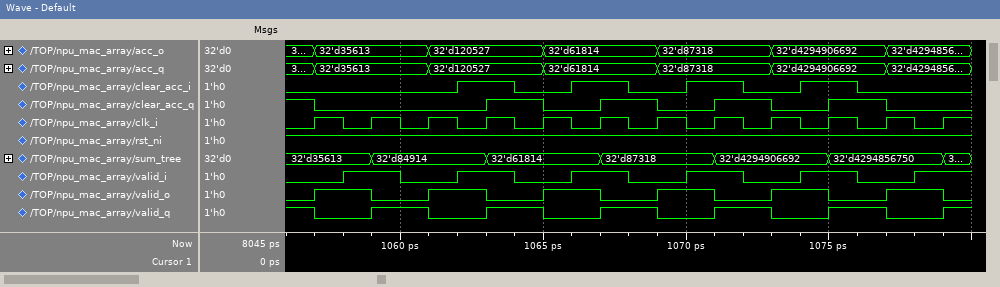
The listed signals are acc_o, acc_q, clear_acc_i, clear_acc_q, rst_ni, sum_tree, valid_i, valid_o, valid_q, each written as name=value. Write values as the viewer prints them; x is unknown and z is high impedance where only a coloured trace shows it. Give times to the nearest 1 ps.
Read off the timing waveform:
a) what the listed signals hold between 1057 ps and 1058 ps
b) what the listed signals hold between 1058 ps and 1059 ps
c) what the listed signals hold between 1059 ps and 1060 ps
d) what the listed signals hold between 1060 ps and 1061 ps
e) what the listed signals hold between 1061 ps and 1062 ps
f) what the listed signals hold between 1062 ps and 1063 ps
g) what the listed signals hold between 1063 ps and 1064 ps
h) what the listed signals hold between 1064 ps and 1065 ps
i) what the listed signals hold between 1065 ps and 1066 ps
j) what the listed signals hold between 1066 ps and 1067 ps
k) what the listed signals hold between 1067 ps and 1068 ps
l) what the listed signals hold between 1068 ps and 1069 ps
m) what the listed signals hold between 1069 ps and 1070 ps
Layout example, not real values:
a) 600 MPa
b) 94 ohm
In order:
a) acc_o=32'd35613, acc_q=32'd35613, clear_acc_i=0, clear_acc_q=0, rst_ni=1, sum_tree=32'd35613, valid_i=0, valid_o=1, valid_q=0
b) acc_o=32'd35613, acc_q=32'd35613, clear_acc_i=0, clear_acc_q=0, rst_ni=1, sum_tree=32'd35613, valid_i=1, valid_o=1, valid_q=0
c) acc_o=32'd35613, acc_q=32'd35613, clear_acc_i=0, clear_acc_q=0, rst_ni=1, sum_tree=32'd84914, valid_i=1, valid_o=0, valid_q=1
d) acc_o=32'd35613, acc_q=32'd35613, clear_acc_i=0, clear_acc_q=0, rst_ni=1, sum_tree=32'd84914, valid_i=0, valid_o=0, valid_q=1
e) acc_o=32'd120527, acc_q=32'd120527, clear_acc_i=0, clear_acc_q=0, rst_ni=1, sum_tree=32'd84914, valid_i=0, valid_o=1, valid_q=0
f) acc_o=32'd120527, acc_q=32'd120527, clear_acc_i=1, clear_acc_q=0, rst_ni=1, sum_tree=32'd84914, valid_i=1, valid_o=1, valid_q=0
g) acc_o=32'd120527, acc_q=32'd120527, clear_acc_i=1, clear_acc_q=1, rst_ni=1, sum_tree=32'd61814, valid_i=1, valid_o=0, valid_q=1
h) acc_o=32'd120527, acc_q=32'd120527, clear_acc_i=0, clear_acc_q=1, rst_ni=1, sum_tree=32'd61814, valid_i=0, valid_o=0, valid_q=1
i) acc_o=32'd61814, acc_q=32'd61814, clear_acc_i=0, clear_acc_q=0, rst_ni=1, sum_tree=32'd61814, valid_i=0, valid_o=1, valid_q=0
j) acc_o=32'd61814, acc_q=32'd61814, clear_acc_i=1, clear_acc_q=0, rst_ni=1, sum_tree=32'd61814, valid_i=1, valid_o=1, valid_q=0
k) acc_o=32'd61814, acc_q=32'd61814, clear_acc_i=1, clear_acc_q=1, rst_ni=1, sum_tree=32'd87318, valid_i=1, valid_o=0, valid_q=1
l) acc_o=32'd61814, acc_q=32'd61814, clear_acc_i=0, clear_acc_q=1, rst_ni=1, sum_tree=32'd87318, valid_i=0, valid_o=0, valid_q=1
m) acc_o=32'd87318, acc_q=32'd87318, clear_acc_i=0, clear_acc_q=0, rst_ni=1, sum_tree=32'd87318, valid_i=0, valid_o=1, valid_q=0
